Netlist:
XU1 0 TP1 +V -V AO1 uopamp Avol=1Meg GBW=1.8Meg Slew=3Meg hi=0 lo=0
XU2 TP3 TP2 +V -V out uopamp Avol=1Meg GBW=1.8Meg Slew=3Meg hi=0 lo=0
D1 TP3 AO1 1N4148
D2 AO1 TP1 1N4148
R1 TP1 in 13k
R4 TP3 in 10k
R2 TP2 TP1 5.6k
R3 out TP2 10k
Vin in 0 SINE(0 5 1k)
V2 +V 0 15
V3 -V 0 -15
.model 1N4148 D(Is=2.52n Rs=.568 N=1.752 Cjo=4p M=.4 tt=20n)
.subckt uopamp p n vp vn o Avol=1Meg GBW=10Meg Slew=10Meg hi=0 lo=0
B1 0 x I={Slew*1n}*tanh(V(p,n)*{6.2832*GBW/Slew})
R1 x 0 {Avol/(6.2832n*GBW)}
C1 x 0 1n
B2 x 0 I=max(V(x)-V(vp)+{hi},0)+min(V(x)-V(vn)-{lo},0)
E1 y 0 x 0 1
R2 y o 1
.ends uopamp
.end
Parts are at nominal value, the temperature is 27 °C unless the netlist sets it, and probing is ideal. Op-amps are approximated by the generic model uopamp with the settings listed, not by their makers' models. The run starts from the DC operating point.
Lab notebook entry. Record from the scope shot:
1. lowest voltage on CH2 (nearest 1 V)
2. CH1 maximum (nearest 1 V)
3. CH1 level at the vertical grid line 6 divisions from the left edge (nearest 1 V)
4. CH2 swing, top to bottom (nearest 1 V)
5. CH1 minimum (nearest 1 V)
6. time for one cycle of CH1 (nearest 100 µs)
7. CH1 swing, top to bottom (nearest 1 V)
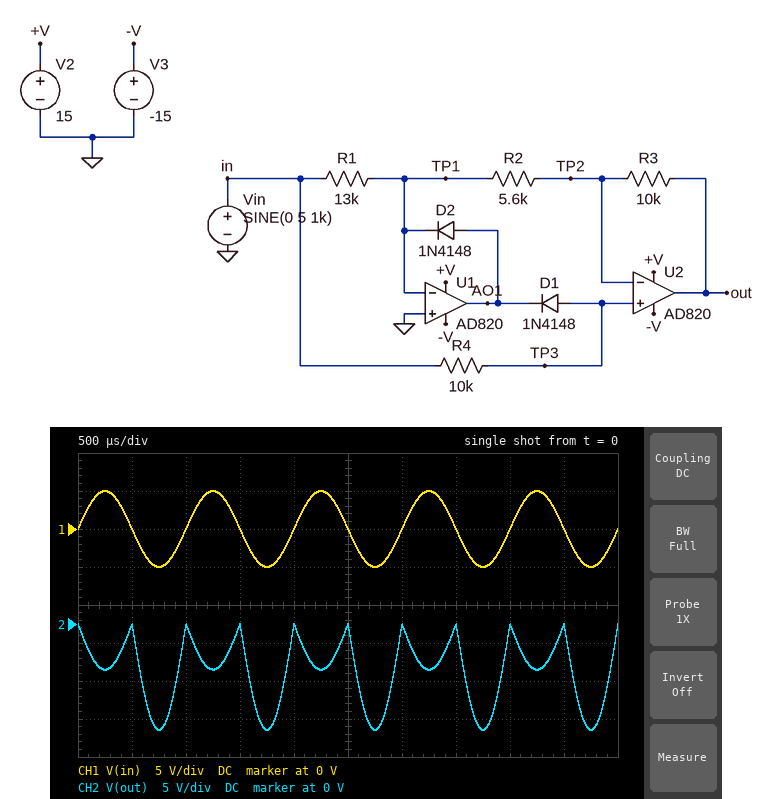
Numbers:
-14 V
5 V
0 V
14 V
-5 V
1.0 ms
10 V
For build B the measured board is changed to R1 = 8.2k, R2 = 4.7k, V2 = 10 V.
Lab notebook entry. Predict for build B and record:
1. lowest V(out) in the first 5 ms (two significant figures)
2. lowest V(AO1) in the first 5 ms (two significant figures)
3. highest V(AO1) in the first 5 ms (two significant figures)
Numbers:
-15 V
-3.4 V
610 mV
